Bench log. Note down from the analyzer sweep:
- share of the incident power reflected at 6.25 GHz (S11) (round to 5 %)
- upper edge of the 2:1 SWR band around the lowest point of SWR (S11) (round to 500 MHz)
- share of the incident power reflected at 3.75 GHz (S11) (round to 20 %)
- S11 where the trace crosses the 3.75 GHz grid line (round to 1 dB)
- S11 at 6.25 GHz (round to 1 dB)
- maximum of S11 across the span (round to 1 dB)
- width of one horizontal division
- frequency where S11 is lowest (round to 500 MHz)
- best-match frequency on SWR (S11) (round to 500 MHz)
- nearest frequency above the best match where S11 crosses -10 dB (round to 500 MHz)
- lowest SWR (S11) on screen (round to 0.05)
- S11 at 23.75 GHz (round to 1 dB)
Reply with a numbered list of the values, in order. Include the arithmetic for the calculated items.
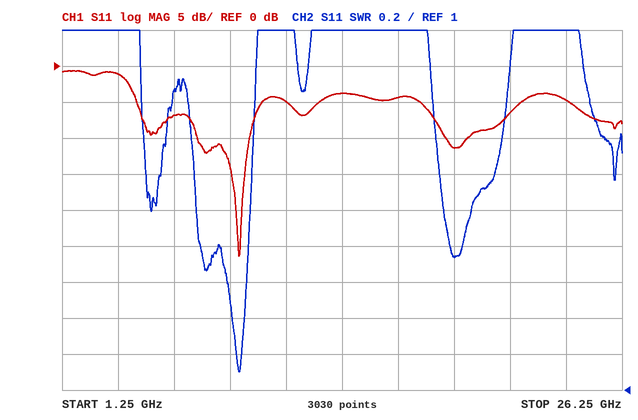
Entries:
1. 10^(-7/10) ≈ 20 %
2. 9.5 GHz
3. 10^(-1/10) ≈ 79.4 %, so 80 % to the nearest 20 %
4. -1 dB
5. -7 dB
6. -1 dB
7. 2.5 GHz
8. 9.0 GHz
9. 9.0 GHz
10. 9.5 GHz
11. 1.10
12. -5 dB
